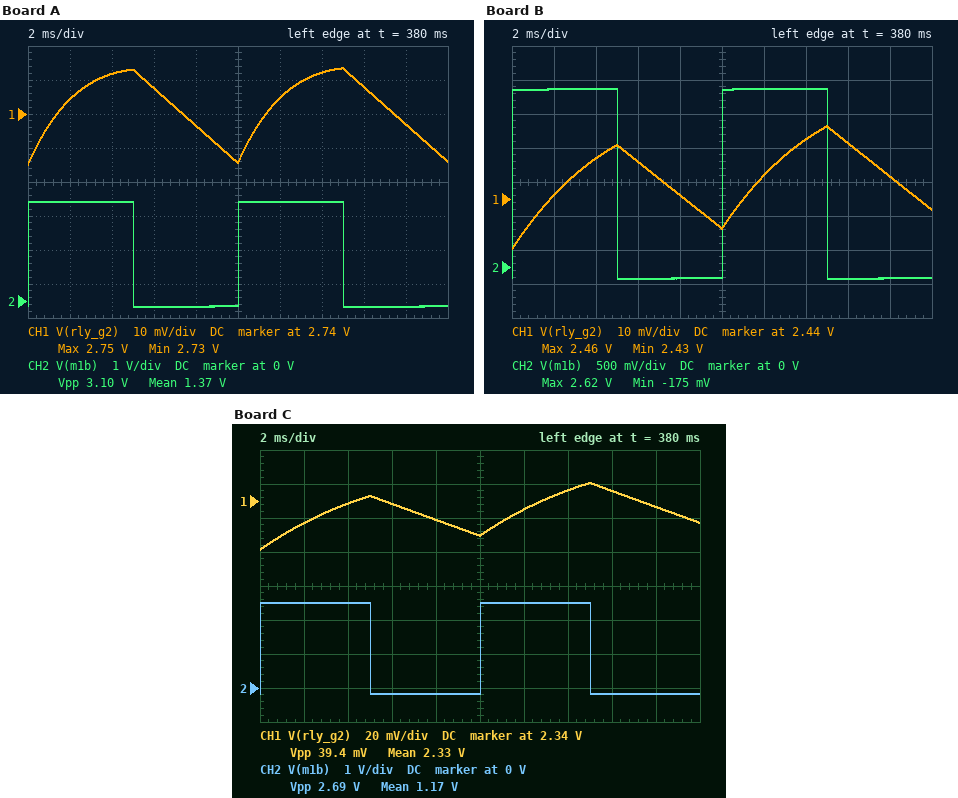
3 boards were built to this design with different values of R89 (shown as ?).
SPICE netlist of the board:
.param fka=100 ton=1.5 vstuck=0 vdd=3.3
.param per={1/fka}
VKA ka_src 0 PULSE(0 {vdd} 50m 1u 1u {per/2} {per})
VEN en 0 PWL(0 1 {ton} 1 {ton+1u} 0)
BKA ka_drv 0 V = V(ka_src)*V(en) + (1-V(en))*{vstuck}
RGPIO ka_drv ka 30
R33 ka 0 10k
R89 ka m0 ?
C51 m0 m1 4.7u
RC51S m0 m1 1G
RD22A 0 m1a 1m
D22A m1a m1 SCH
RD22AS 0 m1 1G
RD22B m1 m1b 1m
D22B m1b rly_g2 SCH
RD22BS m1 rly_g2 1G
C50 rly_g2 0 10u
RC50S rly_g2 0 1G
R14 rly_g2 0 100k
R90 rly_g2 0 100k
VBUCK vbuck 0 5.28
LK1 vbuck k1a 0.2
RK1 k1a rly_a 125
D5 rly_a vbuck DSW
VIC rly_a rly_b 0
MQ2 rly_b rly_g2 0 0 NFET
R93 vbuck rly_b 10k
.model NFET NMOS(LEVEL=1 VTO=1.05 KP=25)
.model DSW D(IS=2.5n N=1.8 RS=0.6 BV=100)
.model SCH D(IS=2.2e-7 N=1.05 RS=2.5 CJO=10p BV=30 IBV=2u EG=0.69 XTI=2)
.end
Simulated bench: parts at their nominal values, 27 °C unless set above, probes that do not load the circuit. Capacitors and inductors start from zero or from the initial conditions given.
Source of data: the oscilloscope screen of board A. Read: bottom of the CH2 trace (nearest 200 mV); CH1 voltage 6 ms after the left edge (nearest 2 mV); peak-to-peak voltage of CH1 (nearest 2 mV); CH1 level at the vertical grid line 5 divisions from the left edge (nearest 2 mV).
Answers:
-200 mV
2.748 V
28 mV
2.726 V
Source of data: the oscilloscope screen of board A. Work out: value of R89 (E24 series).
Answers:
820 Ω
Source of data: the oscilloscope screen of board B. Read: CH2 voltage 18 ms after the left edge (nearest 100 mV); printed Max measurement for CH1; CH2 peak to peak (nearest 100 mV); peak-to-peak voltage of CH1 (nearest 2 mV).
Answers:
-200 mV
2.46 V
2.8 V
36 mV
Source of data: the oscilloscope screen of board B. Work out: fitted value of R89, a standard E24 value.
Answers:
2.2 kΩ
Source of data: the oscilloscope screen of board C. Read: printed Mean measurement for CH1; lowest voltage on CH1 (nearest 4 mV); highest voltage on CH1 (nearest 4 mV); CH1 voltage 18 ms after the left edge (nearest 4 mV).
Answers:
2.33 V
2.312 V
2.352 V
2.336 V
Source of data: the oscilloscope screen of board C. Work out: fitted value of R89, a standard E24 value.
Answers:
2.7 kΩ
